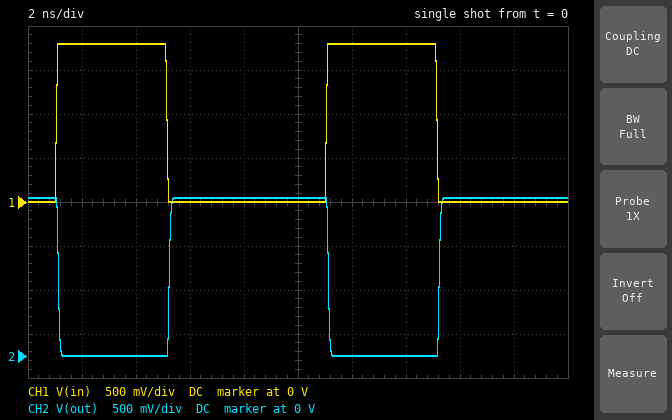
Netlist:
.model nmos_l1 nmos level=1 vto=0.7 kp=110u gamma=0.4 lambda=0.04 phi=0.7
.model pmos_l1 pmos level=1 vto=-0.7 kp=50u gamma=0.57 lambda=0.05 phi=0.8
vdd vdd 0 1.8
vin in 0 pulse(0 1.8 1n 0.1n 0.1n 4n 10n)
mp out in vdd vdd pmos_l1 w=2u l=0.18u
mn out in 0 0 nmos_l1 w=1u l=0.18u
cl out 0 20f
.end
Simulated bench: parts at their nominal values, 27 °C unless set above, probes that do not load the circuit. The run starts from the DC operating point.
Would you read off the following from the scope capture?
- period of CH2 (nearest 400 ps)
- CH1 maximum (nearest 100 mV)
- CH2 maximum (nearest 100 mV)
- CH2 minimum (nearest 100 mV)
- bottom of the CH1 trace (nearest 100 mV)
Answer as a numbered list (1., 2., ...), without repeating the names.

1. 10.0 ns
2. 1.8 V
3. 1.8 V
4. 0 V
5. 0 V
